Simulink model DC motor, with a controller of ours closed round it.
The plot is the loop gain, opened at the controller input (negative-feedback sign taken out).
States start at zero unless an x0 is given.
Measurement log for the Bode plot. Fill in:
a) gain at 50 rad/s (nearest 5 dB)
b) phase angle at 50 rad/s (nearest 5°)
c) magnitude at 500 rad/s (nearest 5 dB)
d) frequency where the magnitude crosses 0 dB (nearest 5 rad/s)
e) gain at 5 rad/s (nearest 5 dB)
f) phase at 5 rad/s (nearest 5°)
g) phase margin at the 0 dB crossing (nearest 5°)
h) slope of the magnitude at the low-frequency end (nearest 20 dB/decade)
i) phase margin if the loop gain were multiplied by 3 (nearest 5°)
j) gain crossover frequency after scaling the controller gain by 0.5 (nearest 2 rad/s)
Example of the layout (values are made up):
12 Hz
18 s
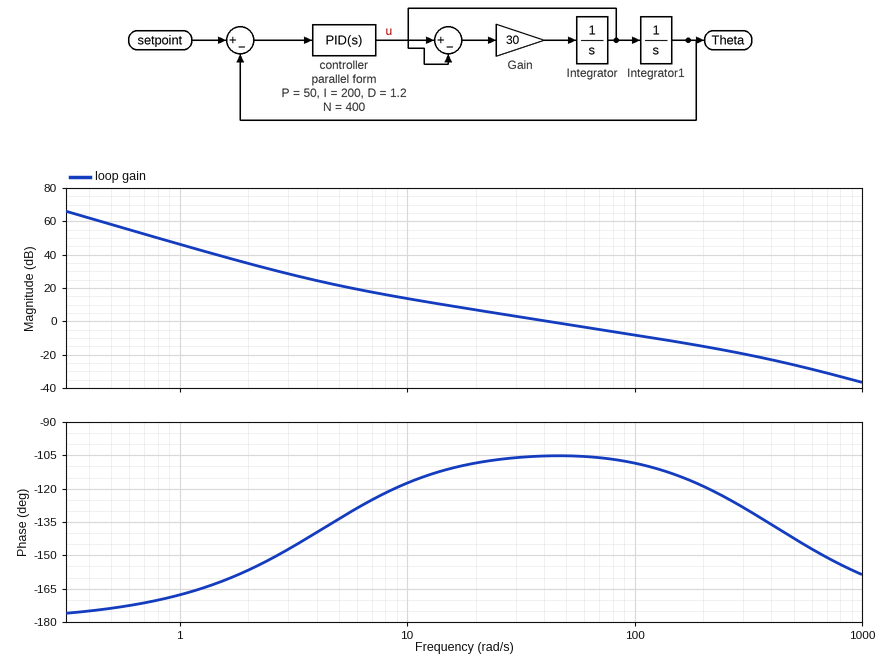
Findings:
0 dB
-105°
-25 dB
40 rad/s
20 dB
-135°
75°
-40 dB/decade
70°
22 rad/s
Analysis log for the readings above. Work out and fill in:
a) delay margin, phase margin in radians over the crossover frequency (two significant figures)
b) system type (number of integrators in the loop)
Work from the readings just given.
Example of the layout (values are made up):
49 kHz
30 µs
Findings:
0.033 s
2
